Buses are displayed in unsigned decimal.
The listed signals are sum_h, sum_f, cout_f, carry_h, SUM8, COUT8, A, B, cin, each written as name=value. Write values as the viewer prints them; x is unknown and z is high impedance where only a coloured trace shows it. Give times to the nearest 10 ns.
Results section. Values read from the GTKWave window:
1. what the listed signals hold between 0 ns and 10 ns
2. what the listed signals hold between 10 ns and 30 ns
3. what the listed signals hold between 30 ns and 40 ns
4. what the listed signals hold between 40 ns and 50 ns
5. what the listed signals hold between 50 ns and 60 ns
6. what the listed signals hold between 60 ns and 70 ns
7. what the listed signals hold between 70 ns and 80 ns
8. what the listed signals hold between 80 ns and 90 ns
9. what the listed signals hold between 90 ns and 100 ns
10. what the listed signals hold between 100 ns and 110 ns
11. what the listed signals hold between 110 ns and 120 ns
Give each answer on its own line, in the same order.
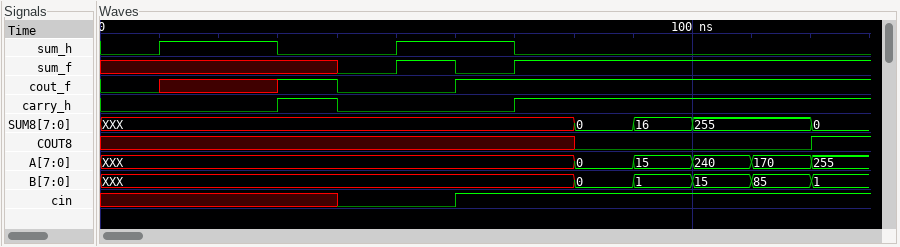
sum_h=0, sum_f=x, cout_f=0, carry_h=0, SUM8=XXX, COUT8=x, A=XXX, B=XXX, cin=x
sum_h=1, sum_f=x, cout_f=x, carry_h=0, SUM8=XXX, COUT8=x, A=XXX, B=XXX, cin=x
sum_h=0, sum_f=x, cout_f=1, carry_h=1, SUM8=XXX, COUT8=x, A=XXX, B=XXX, cin=x
sum_h=0, sum_f=0, cout_f=0, carry_h=0, SUM8=XXX, COUT8=x, A=XXX, B=XXX, cin=0
sum_h=1, sum_f=1, cout_f=0, carry_h=0, SUM8=XXX, COUT8=x, A=XXX, B=XXX, cin=0
sum_h=1, sum_f=0, cout_f=1, carry_h=0, SUM8=XXX, COUT8=x, A=XXX, B=XXX, cin=1
sum_h=0, sum_f=1, cout_f=1, carry_h=1, SUM8=XXX, COUT8=x, A=XXX, B=XXX, cin=1
sum_h=0, sum_f=1, cout_f=1, carry_h=1, SUM8=0, COUT8=0, A=0, B=0, cin=1
sum_h=0, sum_f=1, cout_f=1, carry_h=1, SUM8=16, COUT8=0, A=15, B=1, cin=1
sum_h=0, sum_f=1, cout_f=1, carry_h=1, SUM8=255, COUT8=0, A=240, B=15, cin=1
sum_h=0, sum_f=1, cout_f=1, carry_h=1, SUM8=255, COUT8=0, A=170, B=85, cin=1
